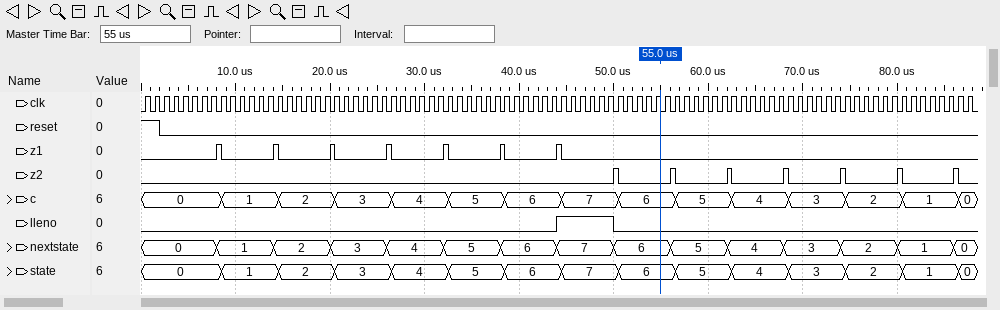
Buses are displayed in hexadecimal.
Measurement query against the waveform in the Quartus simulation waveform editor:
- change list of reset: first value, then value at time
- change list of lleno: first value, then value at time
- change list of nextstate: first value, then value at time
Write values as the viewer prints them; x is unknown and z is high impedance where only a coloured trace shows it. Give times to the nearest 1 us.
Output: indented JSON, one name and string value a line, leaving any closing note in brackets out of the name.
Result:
{
  "change list of reset: first value, then value at time": "1, 0 at 2 us",
  "change list of lleno: first value, then value at time": "0, 1 at 44 us, 0 at 50 us",
  "change list of nextstate: first value, then value at time": "0, 1 at 8 us, 2 at 14 us, 3 at 20 us, 4 at 26 us, 5 at 32 us, 6 at 38 us, 7 at 44 us, 6 at 50 us, 5 at 56 us, 4 at 62 us, 3 at 68 us, 2 at 74 us, 1 at 80 us, 0 at 86 us"
}
